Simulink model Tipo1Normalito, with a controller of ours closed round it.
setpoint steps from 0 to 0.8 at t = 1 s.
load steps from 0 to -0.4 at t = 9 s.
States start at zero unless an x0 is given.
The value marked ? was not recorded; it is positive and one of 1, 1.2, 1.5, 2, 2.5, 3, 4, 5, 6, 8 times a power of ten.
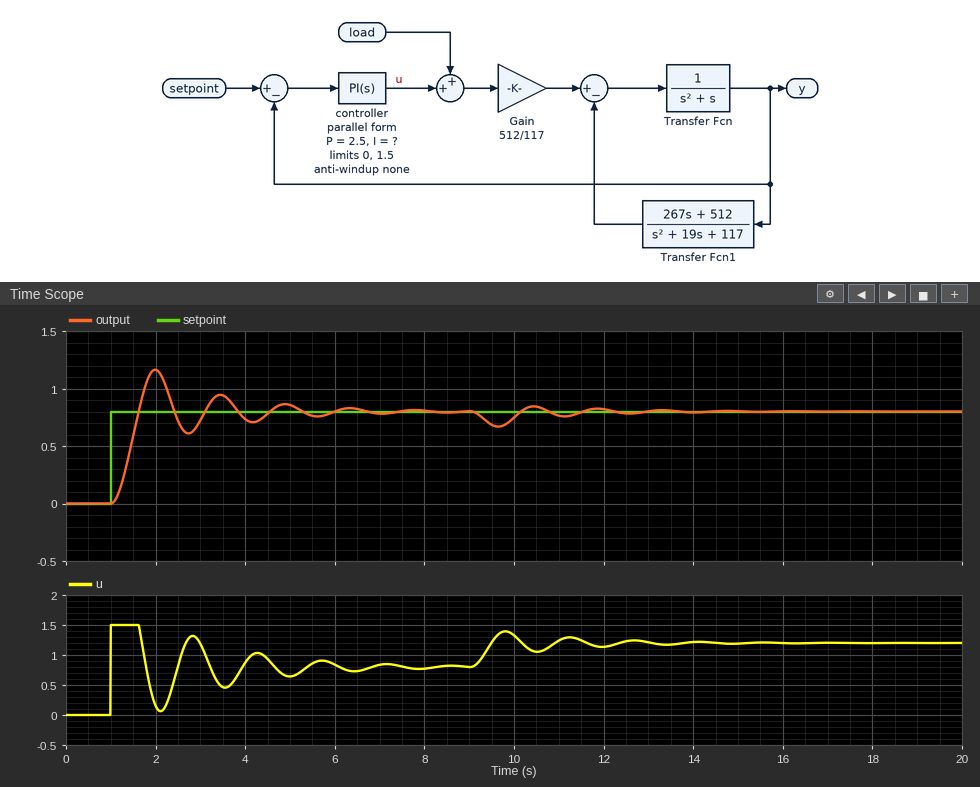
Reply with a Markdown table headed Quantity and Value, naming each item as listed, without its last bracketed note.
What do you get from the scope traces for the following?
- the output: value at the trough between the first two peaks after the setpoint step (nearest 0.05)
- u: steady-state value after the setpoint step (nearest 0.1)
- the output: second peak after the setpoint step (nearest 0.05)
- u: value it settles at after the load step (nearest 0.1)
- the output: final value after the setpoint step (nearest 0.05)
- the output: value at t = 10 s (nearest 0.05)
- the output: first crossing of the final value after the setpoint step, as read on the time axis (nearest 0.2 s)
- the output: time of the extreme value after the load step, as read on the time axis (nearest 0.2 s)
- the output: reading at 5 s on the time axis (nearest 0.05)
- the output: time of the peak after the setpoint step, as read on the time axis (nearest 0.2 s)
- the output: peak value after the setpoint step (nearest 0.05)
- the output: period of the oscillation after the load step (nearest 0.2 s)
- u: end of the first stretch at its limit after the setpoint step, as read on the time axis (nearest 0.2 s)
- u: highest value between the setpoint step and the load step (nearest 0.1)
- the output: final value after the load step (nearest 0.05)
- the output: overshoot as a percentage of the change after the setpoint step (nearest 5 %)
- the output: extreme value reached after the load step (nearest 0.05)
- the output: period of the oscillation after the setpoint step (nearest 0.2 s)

| Quantity | Value |
|---|---|
| the output: value at the trough between the first two peaks after the setpoint step | 0.60 |
| u: steady-state value after the setpoint step | 0.8 |
| the output: second peak after the setpoint step | 0.95 |
| u: value it settles at after the load step | 1.2 |
| the output: final value after the setpoint step | 0.80 |
| the output: value at t = 10 s | 0.75 |
| the output: first crossing of the final value after the setpoint step, as read on the time axis | 1.6 s |
| the output: time of the extreme value after the load step, as read on the time axis | 9.6 s |
| the output: reading at 5 s on the time axis | 0.85 |
| the output: time of the peak after the setpoint step, as read on the time axis | 2.0 s |
| the output: peak value after the setpoint step | 1.15 |
| the output: period of the oscillation after the load step | 1.4 s |
| u: end of the first stretch at its limit after the setpoint step, as read on the time axis | 1.6 s |
| u: highest value between the setpoint step and the load step | 1.5 |
| the output: final value after the load step | 0.80 |
| the output: overshoot as a percentage of the change after the setpoint step | 45 % |
| the output: extreme value reached after the load step | 0.65 |
| the output: period of the oscillation after the setpoint step | 1.4 s |
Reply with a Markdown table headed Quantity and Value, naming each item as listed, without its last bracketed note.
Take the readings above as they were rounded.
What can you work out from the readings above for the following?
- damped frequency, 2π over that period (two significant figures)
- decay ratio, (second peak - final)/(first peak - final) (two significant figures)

| Quantity | Value |
|---|---|
| damped frequency, 2π over that period | 4.5 rad/s |
| decay ratio, (second peak - final)/(first peak - final) | 0.43 |
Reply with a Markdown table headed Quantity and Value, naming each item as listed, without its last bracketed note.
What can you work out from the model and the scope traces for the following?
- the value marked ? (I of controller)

| Quantity | Value |
|---|---|
| the value marked ? | 5 |
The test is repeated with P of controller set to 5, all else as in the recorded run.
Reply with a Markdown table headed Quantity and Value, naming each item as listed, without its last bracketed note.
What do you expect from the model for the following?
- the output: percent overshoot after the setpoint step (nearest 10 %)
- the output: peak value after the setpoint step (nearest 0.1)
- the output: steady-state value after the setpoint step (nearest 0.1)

| Quantity | Value |
|---|---|
| the output: percent overshoot after the setpoint step | 40 % |
| the output: peak value after the setpoint step | 1.1 |
| the output: steady-state value after the setpoint step | 0.8 |
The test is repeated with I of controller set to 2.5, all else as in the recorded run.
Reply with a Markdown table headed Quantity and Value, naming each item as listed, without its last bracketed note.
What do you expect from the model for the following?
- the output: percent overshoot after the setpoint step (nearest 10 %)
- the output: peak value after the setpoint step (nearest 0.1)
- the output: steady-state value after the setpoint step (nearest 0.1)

| Quantity | Value |
|---|---|
| the output: percent overshoot after the setpoint step | 20 % |
| the output: peak value after the setpoint step | 1.0 |
| the output: steady-state value after the setpoint step | 0.8 |
